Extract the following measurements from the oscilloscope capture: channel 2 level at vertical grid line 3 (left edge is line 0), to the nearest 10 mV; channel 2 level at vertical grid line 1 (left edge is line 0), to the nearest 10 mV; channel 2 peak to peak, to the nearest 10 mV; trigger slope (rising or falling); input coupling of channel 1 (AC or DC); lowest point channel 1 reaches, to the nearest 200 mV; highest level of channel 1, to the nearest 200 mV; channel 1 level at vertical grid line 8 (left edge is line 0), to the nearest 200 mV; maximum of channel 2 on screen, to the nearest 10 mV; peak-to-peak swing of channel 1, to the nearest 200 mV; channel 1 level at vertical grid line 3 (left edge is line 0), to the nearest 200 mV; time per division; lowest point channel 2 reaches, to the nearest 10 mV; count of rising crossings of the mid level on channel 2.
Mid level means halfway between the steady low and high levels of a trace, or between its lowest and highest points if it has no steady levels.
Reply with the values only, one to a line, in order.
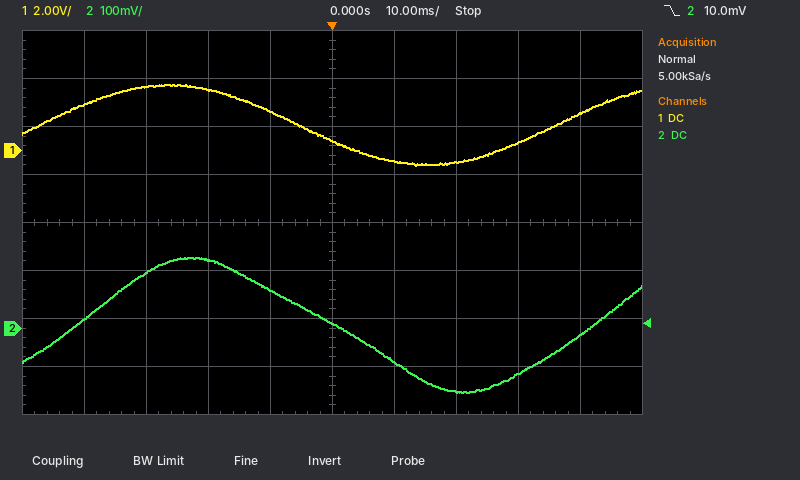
140 mV
20 mV
280 mV
falling
DC
-600 mV
2.8 V
400 mV
150 mV
3.4 V
2.6 V
10 ms
-130 mV
2
